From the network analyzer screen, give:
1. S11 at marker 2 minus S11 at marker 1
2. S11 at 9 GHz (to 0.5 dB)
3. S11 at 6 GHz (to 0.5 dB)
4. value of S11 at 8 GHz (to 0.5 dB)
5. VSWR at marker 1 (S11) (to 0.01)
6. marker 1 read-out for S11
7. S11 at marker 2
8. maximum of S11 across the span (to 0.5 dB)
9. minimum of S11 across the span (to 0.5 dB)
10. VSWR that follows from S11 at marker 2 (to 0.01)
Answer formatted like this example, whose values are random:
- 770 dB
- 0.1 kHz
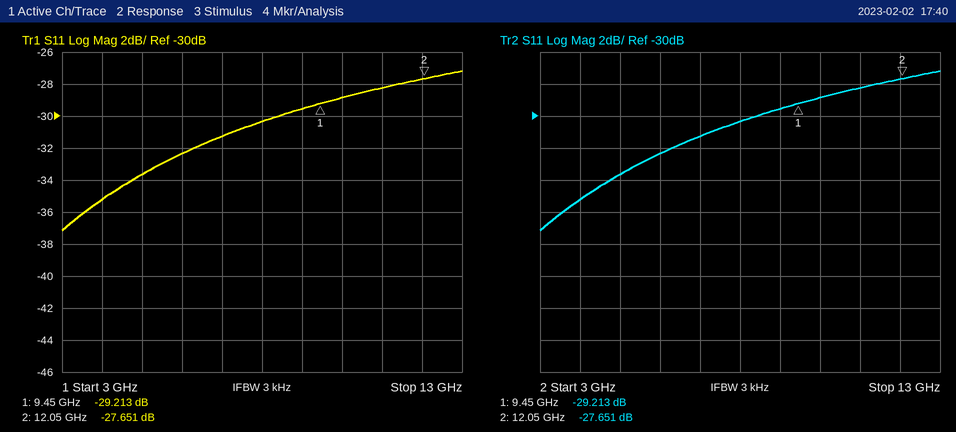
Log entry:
- 1.562 dB
- -29.5 dB
- -32.5 dB
- -30.5 dB
- 1.07
- -29.213 dB
- -27.651 dB
- -27.0 dB
- -37.0 dB
- 1.09
